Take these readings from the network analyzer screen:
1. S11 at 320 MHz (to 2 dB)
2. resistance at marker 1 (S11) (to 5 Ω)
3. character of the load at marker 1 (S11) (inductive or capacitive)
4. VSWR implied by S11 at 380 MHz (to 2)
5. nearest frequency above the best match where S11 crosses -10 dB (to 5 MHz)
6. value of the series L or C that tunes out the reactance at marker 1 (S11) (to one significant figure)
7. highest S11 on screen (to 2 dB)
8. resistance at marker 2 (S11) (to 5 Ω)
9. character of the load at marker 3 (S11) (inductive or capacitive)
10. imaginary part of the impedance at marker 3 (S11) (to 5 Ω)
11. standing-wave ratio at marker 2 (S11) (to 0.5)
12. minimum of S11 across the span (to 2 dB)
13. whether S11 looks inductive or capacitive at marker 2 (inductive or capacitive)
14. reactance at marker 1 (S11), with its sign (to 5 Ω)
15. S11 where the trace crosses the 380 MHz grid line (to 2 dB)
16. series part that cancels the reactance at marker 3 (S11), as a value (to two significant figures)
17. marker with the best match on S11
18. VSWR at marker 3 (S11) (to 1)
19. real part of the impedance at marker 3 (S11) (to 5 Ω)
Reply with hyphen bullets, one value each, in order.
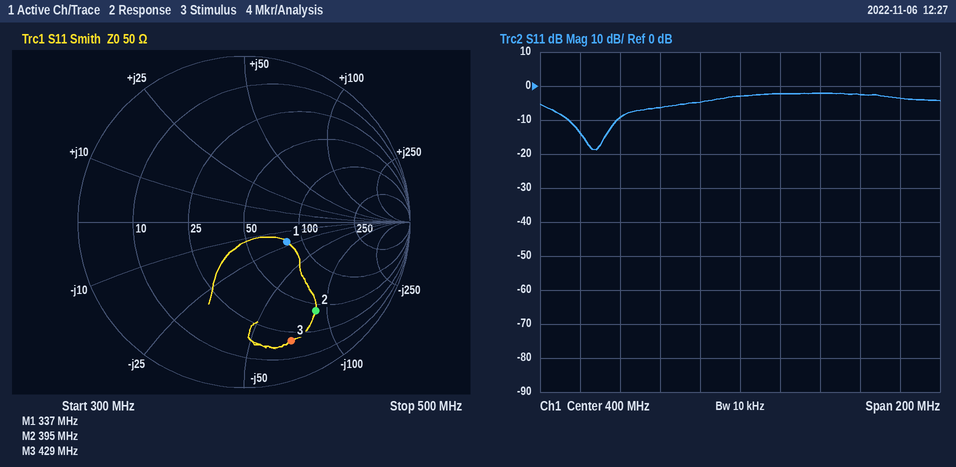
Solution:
- -14 dB
- 80 Ω
- capacitive
- 4
- 340 MHz
- 10 nH
- -2 dB
- 45 Ω
- capacitive
- -70 Ω
- 5.5
- -18 dB
- capacitive
- -20 Ω
- -4 dB
- 26 nH
- marker 1
- 8
- 20 Ω
